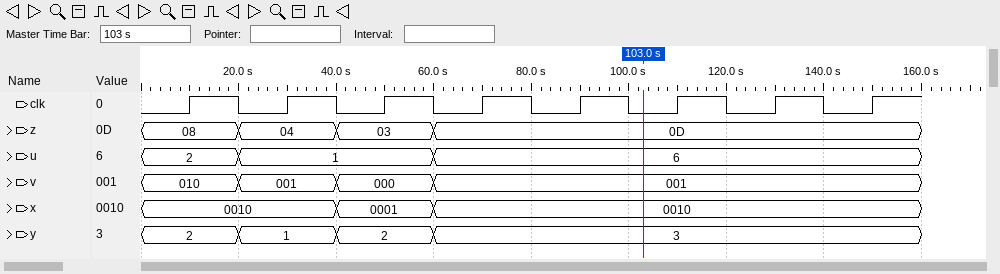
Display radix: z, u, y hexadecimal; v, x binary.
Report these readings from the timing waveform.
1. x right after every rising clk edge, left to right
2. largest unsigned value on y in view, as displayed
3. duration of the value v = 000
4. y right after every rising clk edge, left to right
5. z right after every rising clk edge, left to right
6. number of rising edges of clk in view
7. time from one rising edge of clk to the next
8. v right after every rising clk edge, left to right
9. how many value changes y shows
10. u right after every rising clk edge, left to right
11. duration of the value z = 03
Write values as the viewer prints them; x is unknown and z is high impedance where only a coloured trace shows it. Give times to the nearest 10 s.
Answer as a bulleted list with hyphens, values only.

- 0010, 0010, 0001, 0010, 0010, 0010, 0010, 0010
- 3
- 20 s
- 2, 1, 2, 3, 3, 3, 3, 3
- 08, 04, 03, 0D, 0D, 0D, 0D, 0D
- 8
- 20 s
- 010, 001, 000, 001, 001, 001, 001, 001
- 3
- 2, 1, 1, 6, 6, 6, 6, 6
- 20 s
